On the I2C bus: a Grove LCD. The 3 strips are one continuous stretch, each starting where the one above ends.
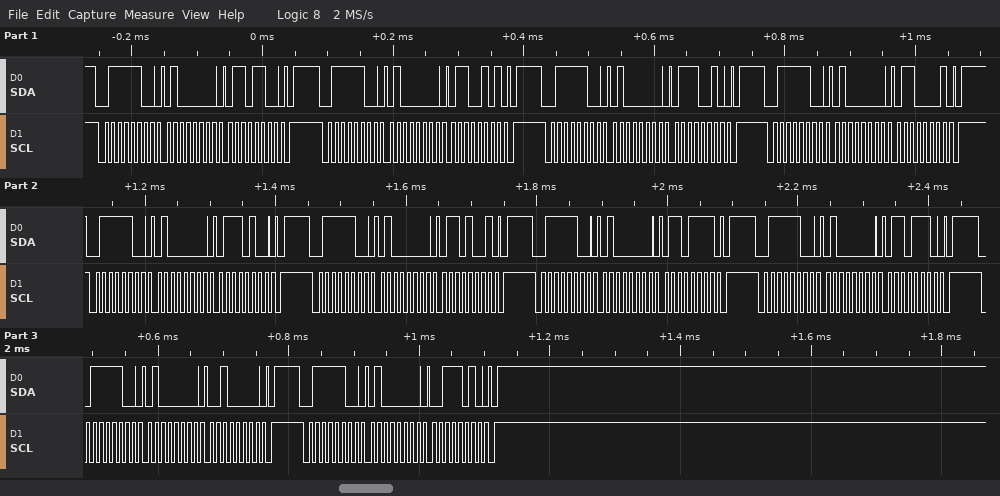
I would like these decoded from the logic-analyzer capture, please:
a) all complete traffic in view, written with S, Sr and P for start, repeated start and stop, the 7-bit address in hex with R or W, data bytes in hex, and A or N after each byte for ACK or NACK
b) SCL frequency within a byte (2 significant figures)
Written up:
S 3EW A 40 A 6C A P S 3EW A 40 A 65 A P S 3EW A 40 A 72 A P S 3EW A 40 A 61 A P S 3EW A 40 A 74 A P S 3EW A 40 A 69 A P S 3EW A 40 A 6F A P S 3EW A 40 A 6E A P S 3EW A 40 A 20 A P S 3EW A 40 A 3A A P
100 kHz
